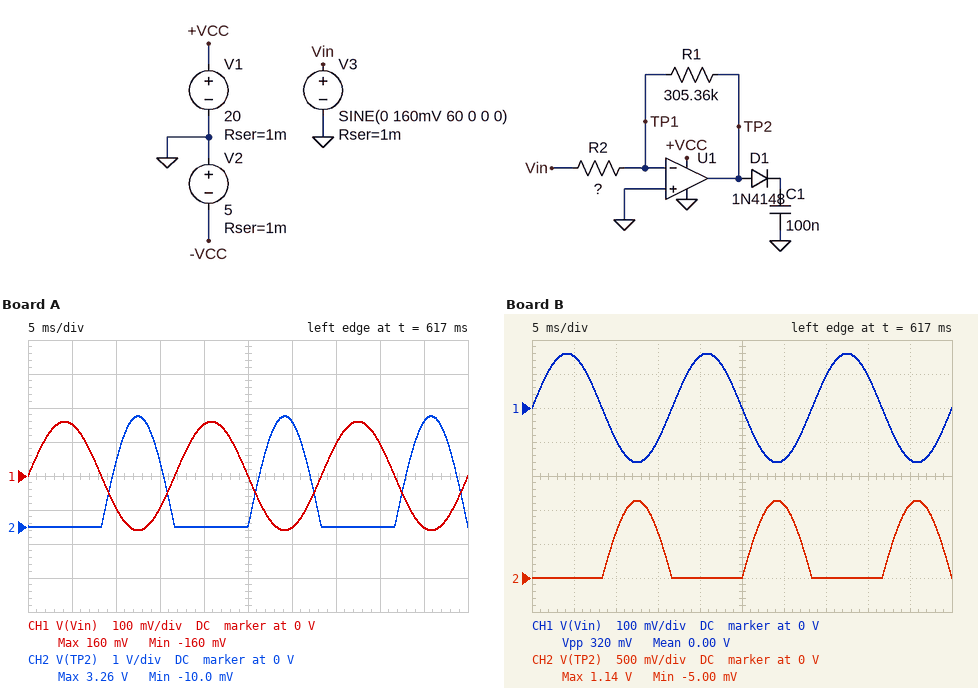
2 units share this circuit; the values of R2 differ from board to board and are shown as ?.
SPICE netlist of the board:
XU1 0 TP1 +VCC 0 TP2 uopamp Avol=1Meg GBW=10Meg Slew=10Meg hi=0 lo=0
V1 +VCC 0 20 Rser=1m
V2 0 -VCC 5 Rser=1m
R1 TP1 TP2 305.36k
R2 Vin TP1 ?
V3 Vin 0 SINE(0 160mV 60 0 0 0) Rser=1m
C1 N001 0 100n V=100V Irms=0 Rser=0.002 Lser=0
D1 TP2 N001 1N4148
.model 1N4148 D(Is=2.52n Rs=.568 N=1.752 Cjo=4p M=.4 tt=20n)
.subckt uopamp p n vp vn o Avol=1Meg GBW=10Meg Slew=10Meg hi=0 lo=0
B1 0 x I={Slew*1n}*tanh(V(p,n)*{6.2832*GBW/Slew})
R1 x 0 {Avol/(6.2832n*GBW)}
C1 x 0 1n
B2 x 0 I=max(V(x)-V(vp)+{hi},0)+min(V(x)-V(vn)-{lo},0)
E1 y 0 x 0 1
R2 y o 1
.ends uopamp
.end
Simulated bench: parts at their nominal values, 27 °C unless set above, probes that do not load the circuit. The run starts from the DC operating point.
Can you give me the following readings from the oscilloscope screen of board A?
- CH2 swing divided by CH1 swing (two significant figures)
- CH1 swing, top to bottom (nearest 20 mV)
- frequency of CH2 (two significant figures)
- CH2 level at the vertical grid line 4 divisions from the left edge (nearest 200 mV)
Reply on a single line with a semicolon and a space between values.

10; 320 mV; 60 Hz; 0 V
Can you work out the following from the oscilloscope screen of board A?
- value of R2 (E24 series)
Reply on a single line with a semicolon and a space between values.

15 kΩ
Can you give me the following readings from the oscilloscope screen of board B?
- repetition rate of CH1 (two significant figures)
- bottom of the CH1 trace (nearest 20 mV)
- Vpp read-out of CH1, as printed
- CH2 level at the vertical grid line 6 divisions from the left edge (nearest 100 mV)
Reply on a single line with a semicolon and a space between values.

60 Hz; -160 mV; 320 mV; 1.1 V
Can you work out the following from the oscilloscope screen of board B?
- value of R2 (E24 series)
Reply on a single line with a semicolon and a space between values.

43 kΩ
